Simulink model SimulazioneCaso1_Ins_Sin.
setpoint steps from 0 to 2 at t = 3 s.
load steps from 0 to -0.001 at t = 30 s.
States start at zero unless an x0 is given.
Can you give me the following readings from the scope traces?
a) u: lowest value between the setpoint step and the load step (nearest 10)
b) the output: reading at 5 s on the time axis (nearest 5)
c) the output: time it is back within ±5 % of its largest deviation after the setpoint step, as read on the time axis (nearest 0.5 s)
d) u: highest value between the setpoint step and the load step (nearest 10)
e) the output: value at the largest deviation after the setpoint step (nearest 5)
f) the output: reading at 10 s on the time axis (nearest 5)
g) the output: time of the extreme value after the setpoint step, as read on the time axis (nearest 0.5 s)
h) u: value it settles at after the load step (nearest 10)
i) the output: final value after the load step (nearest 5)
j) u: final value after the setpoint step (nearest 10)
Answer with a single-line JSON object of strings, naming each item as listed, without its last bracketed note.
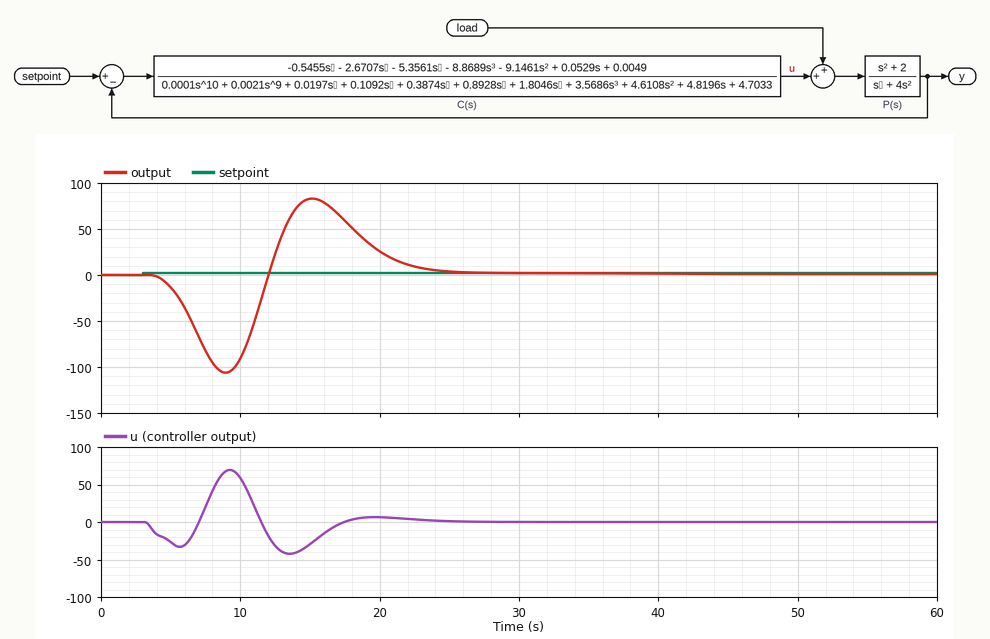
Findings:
{"u: lowest value between the setpoint step and the load step": "-40", "the output: reading at 5 s on the time axis": "-15", "the output: time it is back within ±5 % of its largest deviation after the setpoint step, as read on the time axis": "23.0 s", "u: highest value between the setpoint step and the load step": "70", "the output: value at the largest deviation after the setpoint step": "-105", "the output: reading at 10 s on the time axis": "-90", "the output: time of the extreme value after the setpoint step, as read on the time axis": "9.0 s", "u: value it settles at after the load step": "0", "the output: final value after the load step": "0", "u: final value after the setpoint step": "0"}
